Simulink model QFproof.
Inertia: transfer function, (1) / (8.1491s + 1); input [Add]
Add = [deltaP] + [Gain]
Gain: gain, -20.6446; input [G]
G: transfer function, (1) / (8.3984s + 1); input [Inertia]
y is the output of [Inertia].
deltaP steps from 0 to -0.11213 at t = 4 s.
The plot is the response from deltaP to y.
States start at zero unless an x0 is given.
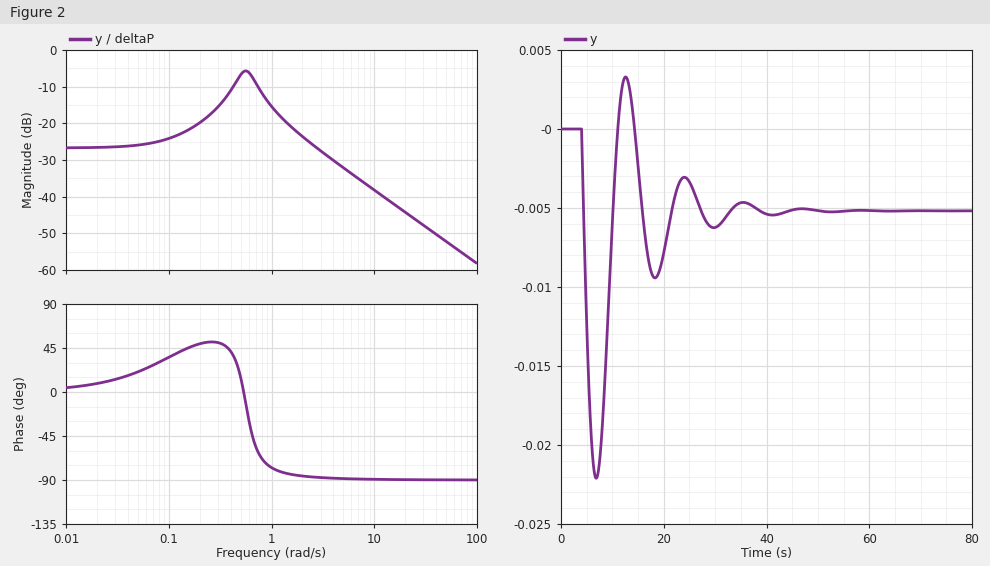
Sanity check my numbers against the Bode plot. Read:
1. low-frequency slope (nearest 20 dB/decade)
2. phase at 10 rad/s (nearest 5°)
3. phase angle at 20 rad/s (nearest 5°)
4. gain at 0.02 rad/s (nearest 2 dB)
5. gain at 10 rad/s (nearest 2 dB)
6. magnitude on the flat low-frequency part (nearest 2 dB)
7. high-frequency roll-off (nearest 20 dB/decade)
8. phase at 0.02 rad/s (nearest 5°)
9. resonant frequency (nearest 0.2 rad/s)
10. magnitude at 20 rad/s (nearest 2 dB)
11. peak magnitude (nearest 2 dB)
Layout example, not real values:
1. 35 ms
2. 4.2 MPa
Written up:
1. 0 dB/decade
2. -90°
3. -90°
4. -26 dB
5. -38 dB
6. -26 dB
7. -20 dB/decade
8. 10°
9. 0.6 rad/s
10. -44 dB
11. -6 dB
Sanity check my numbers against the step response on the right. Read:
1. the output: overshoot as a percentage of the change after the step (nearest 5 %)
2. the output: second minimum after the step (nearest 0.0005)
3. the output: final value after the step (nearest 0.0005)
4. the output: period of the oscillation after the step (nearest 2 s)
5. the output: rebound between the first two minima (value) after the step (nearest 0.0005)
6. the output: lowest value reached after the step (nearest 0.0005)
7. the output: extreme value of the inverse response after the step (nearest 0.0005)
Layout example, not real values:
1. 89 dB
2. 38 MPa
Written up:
1. 325 %
2. -0.0095
3. -0.0050
4. 12 s
5. 0.0035
6. -0.0220
7. 0.0035
